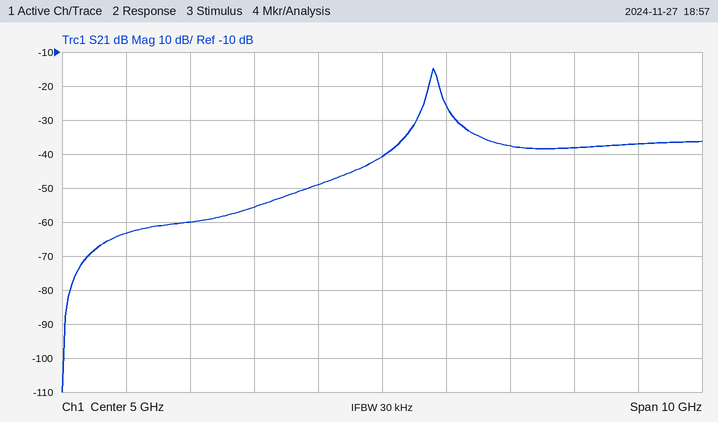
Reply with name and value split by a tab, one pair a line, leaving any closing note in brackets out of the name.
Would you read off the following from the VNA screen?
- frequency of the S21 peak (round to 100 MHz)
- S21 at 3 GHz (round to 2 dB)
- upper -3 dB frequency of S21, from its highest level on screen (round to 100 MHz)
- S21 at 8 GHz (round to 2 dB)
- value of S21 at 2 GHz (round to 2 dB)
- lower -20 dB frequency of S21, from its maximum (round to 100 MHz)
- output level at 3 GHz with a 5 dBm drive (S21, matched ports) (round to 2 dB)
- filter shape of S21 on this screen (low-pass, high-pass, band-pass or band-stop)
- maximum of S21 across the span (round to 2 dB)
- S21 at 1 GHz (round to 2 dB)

frequency of the S21 peak	5.8 GHz
S21 at 3 GHz	-56 dB
upper -3 dB frequency of S21, from its highest level on screen	5.9 GHz
S21 at 8 GHz	-38 dB
value of S21 at 2 GHz	-60 dB
lower -20 dB frequency of S21, from its maximum	5.4 GHz
output level at 3 GHz with a 5 dBm drive (S21, matched ports)	-50 dBm
filter shape of S21 on this screen	band-pass
maximum of S21 across the span	-14 dB
S21 at 1 GHz	-64 dB
